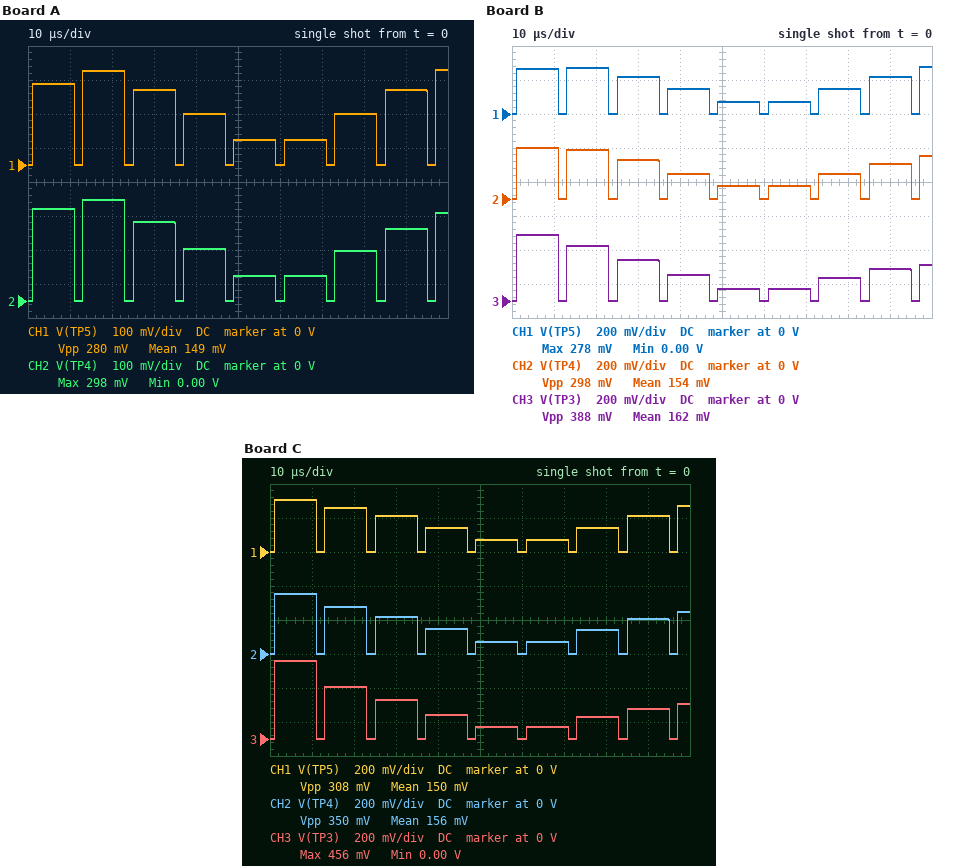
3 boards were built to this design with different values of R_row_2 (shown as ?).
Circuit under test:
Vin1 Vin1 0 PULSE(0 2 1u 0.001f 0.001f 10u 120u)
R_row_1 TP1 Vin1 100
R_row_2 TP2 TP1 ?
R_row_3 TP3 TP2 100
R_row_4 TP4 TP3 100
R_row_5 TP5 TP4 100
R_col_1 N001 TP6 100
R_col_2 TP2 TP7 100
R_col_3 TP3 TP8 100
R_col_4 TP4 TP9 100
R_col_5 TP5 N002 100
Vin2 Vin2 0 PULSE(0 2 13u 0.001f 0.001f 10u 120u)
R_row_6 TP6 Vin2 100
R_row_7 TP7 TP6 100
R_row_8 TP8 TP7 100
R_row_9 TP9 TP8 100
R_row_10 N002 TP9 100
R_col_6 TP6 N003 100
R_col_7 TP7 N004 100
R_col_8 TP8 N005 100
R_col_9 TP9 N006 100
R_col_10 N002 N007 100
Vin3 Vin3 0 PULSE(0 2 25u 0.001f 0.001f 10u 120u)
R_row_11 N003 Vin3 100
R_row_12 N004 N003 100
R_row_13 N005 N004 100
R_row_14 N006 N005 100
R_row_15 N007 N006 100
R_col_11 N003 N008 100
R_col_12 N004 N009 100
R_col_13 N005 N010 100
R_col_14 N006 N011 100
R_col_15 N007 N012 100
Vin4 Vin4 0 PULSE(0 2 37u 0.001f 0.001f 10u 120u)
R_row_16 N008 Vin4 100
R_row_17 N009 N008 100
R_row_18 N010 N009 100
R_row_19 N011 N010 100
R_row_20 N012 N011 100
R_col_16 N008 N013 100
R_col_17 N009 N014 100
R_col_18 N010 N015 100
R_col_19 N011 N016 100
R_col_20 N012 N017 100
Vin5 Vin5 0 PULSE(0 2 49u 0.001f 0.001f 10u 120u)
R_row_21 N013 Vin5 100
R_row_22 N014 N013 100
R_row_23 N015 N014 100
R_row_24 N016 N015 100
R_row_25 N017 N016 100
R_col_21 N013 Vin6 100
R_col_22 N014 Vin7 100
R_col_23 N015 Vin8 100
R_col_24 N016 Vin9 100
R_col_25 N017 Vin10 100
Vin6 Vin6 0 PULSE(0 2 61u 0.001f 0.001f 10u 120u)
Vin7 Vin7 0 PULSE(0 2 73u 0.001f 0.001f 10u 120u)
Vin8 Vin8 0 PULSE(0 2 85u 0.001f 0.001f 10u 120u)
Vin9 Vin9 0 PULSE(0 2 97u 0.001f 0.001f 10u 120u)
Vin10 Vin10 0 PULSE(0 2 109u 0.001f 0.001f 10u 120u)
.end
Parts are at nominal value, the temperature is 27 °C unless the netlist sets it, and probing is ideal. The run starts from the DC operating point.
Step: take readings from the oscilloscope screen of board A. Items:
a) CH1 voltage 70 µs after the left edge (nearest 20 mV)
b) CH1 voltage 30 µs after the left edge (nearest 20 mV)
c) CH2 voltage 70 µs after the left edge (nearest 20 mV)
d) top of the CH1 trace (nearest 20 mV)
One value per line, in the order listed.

80 mV
220 mV
80 mV
280 mV
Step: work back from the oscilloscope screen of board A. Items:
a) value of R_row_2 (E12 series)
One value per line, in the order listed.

220 Ω
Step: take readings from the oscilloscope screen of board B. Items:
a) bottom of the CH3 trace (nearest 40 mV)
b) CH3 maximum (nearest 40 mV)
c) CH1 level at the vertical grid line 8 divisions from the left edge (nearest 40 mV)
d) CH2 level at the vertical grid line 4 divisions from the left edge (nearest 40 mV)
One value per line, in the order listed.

0 V
400 mV
160 mV
160 mV
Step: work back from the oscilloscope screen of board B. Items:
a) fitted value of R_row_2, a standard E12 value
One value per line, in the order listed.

180 Ω
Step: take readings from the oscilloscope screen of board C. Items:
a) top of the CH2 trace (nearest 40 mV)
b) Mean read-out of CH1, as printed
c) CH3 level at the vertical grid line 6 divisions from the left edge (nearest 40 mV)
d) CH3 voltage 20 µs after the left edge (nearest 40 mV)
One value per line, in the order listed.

360 mV
150 mV
0 V
320 mV
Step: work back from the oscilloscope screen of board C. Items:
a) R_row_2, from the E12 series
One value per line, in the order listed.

120 Ω
